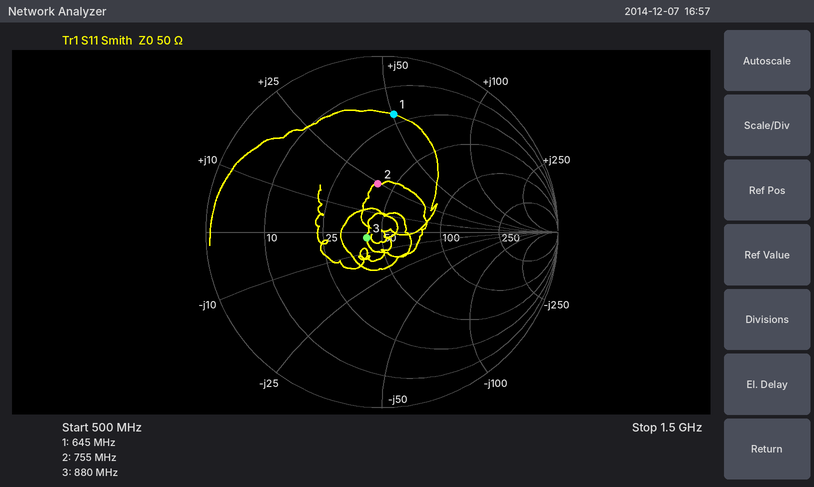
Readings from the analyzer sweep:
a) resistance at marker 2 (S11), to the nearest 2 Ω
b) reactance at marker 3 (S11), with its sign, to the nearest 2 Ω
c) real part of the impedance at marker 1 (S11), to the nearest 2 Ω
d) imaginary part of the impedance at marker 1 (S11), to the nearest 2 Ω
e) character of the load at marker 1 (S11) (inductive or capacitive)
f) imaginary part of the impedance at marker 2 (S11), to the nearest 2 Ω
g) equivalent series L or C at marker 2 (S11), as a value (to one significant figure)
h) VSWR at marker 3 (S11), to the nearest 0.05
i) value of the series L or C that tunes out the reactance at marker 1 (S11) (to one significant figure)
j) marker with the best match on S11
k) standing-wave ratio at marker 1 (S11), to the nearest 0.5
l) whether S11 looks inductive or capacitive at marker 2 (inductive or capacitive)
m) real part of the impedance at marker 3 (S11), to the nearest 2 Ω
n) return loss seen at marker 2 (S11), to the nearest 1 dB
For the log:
42 Ω
-2 Ω
20 Ω
+50 Ω
inductive
+24 Ω
5 nH
1.20
5 pF
marker 3
5.0
inductive
42 Ω
11 dB
